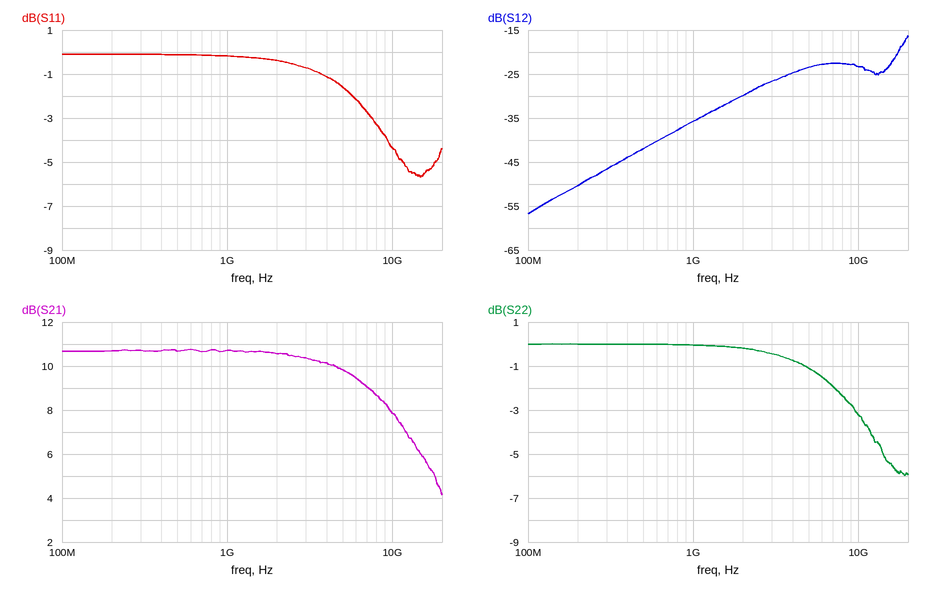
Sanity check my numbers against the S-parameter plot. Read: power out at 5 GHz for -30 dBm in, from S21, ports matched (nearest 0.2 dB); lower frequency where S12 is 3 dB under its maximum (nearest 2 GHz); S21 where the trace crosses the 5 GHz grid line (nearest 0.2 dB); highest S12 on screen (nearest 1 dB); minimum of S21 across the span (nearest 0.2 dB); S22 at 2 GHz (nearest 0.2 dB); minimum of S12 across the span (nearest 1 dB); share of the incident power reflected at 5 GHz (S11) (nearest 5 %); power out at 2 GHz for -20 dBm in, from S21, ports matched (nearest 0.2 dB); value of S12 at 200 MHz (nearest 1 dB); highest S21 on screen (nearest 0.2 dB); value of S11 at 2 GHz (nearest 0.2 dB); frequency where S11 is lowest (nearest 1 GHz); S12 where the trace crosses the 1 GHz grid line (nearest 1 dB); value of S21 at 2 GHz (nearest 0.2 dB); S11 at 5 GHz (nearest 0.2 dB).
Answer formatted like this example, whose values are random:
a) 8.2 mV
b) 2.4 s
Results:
a) -20.2 dBm
b) 18 GHz
c) 9.8 dB
d) -16 dB
e) 4.2 dB
f) -0.2 dB
g) -57 dB
h) 70 %
i) -9.4 dBm
j) -50 dB
k) 10.8 dB
l) -0.4 dB
m) 15 GHz
n) -36 dB
o) 10.6 dB
p) -1.6 dB
